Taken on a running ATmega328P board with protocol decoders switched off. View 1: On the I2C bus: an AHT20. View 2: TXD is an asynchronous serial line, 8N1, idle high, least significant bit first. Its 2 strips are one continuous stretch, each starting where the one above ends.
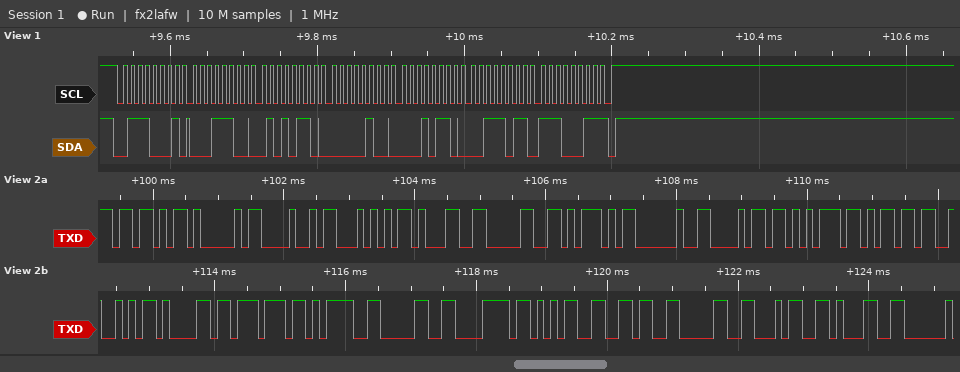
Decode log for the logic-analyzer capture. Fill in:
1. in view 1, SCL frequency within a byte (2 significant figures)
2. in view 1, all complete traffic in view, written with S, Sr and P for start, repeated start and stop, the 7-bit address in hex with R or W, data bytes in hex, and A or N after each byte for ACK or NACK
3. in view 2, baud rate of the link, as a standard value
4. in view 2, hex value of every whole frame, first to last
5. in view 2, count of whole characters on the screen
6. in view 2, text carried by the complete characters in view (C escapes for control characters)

100 kHz
S 38R A 1C A 56 A 04 A 16 A 3B A E3 N P
9600 baud
0x5B 0x41 0x48 0x54 0x31 0x30 0x5D 0x20 0x68 0x75 0x6D 0x52 0x61 0x77 0x3D 0x30 0x78 0x35 0x36 0x30 0x34 0x31
22
"[AHT10] humRaw=0x56041"
